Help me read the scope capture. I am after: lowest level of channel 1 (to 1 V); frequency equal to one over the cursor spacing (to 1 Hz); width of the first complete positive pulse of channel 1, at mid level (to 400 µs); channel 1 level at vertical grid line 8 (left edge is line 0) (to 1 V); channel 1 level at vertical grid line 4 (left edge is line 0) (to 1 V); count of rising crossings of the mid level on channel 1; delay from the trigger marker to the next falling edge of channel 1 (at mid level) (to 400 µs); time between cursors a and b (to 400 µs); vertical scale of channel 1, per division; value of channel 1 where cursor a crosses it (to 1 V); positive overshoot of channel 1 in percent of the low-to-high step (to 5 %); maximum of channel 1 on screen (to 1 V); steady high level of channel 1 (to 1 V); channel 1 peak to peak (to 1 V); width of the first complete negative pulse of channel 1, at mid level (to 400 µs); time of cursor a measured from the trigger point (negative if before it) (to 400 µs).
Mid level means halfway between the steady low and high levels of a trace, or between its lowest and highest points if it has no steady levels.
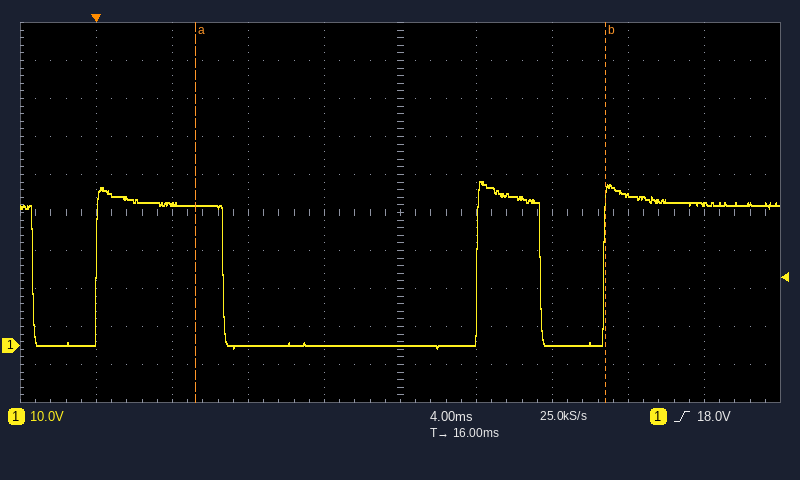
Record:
-1 V
46 Hz
6.8 ms
40 V
0 V
3
6.8 ms
21.6 ms
10 V
37 V
15 %
43 V
37 V
44 V
3.2 ms
+5.2 ms
